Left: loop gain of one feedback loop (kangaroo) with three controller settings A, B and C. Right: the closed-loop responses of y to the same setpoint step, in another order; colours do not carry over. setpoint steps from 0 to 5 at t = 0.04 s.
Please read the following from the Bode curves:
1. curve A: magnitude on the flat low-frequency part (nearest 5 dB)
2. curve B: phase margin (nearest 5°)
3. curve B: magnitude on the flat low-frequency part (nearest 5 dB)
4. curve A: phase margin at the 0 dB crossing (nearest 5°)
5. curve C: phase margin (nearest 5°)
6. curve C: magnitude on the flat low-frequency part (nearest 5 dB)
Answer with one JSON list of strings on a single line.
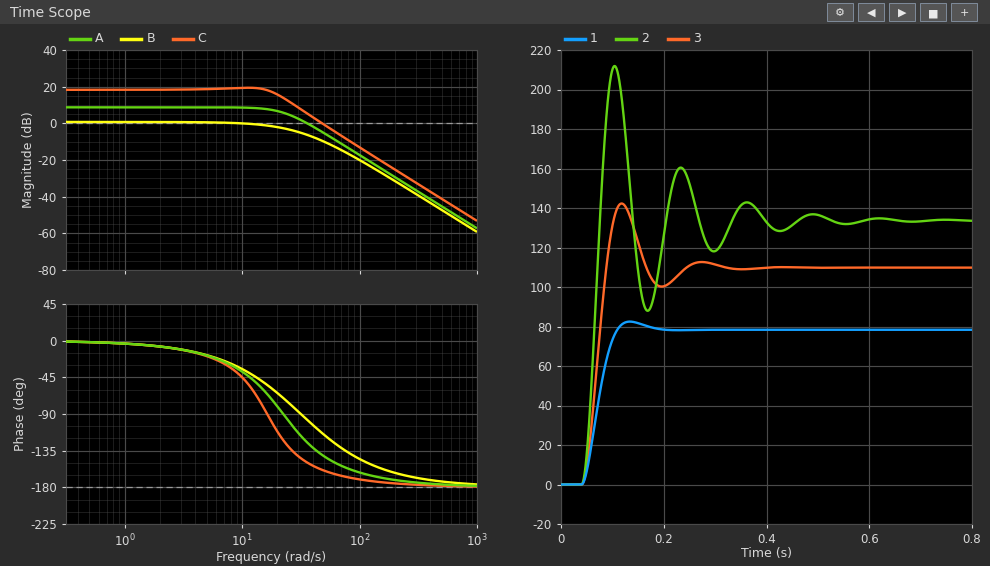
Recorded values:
["10 dB", "145°", "0 dB", "55°", "20°", "20 dB"]
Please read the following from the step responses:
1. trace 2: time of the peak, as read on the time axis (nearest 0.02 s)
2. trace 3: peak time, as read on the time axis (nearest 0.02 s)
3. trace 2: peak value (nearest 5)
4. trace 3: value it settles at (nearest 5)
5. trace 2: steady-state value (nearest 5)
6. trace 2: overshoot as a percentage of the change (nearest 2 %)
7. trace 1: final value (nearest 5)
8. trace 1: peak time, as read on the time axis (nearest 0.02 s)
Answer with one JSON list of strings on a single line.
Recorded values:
["0.10 s", "0.12 s", "210", "110", "135", "58 %", "80", "0.14 s"]
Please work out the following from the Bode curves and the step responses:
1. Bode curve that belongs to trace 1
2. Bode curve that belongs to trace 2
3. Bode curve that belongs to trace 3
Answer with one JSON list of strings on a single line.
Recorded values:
["B", "C", "A"]
